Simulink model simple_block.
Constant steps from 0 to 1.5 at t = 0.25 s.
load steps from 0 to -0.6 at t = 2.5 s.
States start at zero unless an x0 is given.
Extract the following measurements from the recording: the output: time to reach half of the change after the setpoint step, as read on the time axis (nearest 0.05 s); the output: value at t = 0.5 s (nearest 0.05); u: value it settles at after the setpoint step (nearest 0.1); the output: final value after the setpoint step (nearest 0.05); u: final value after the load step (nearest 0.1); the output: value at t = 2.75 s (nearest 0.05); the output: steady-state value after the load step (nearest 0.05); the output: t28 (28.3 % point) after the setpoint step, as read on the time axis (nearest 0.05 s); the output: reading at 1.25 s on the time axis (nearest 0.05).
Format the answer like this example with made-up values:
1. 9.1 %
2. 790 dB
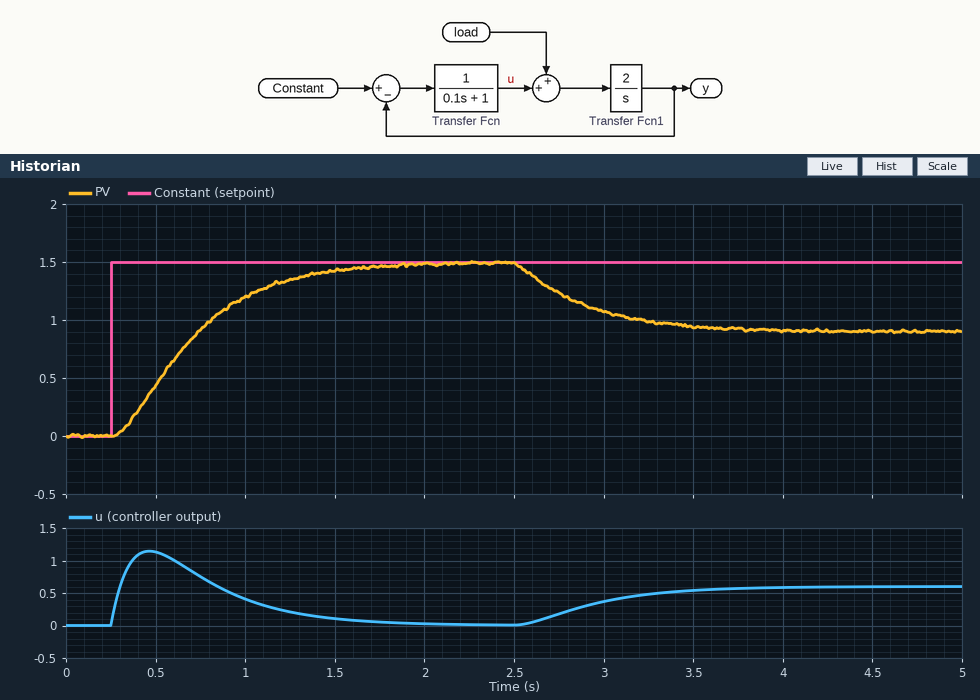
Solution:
1. 0.65 s
2. 0.45
3. 0.0
4. 1.50
5. 0.6
6. 1.25
7. 0.90
8. 0.50 s
9. 1.35
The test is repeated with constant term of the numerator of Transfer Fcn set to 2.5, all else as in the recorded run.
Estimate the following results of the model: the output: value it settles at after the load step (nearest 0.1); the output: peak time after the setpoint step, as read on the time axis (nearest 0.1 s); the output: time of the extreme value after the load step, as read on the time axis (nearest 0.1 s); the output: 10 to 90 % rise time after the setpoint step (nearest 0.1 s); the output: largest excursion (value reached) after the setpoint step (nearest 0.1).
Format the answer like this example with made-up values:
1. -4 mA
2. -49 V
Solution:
1. 1.3
2. 0.9 s
3. 3.0 s
4. 0.3 s
5. 1.6
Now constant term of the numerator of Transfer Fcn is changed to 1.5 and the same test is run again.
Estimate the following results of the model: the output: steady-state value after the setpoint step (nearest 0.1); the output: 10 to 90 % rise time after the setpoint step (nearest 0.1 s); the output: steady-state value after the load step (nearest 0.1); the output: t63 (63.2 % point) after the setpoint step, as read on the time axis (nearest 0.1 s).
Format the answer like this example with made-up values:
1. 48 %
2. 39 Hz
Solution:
1. 1.5
2. 0.5 s
3. 1.1
4. 0.6 s
